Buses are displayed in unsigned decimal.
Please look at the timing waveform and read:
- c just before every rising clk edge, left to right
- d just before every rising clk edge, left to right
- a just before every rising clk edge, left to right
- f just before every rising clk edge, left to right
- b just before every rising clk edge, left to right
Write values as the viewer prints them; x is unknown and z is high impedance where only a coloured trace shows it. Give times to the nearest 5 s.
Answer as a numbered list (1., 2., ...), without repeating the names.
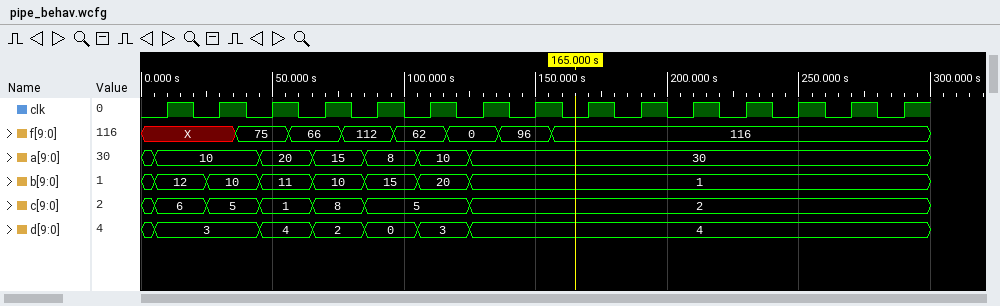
1. 6, 5, 1, 8, 5, 5, 2, 2, 2, 2, 2, 2, 2, 2, 2
2. 3, 3, 4, 2, 0, 3, 4, 4, 4, 4, 4, 4, 4, 4, 4
3. 10, 10, 20, 15, 8, 10, 30, 30, 30, 30, 30, 30, 30, 30, 30
4. X, X, 75, 66, 112, 62, 0, 96, 116, 116, 116, 116, 116, 116, 116
5. 12, 10, 11, 10, 15, 20, 1, 1, 1, 1, 1, 1, 1, 1, 1
